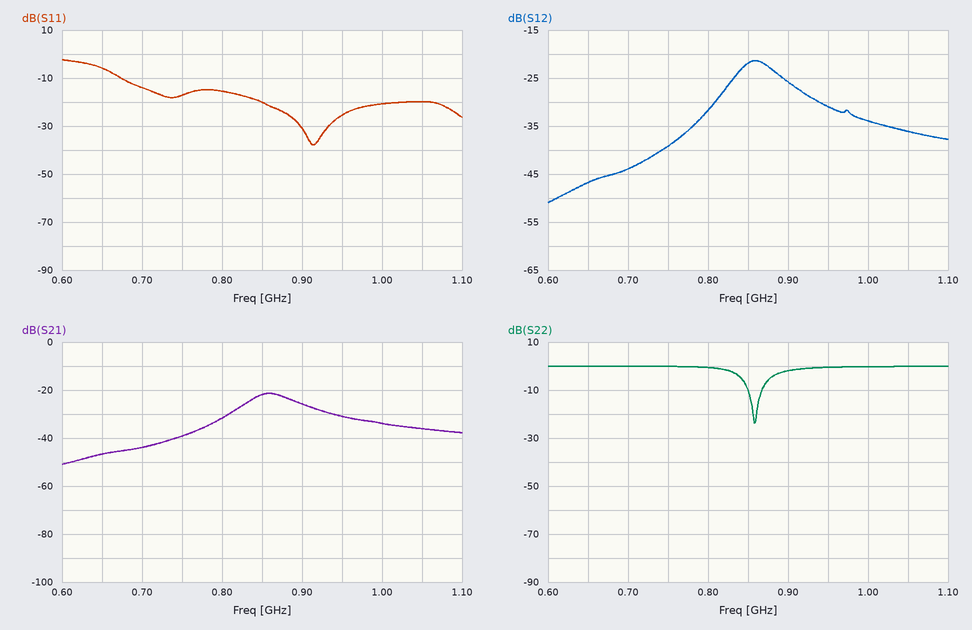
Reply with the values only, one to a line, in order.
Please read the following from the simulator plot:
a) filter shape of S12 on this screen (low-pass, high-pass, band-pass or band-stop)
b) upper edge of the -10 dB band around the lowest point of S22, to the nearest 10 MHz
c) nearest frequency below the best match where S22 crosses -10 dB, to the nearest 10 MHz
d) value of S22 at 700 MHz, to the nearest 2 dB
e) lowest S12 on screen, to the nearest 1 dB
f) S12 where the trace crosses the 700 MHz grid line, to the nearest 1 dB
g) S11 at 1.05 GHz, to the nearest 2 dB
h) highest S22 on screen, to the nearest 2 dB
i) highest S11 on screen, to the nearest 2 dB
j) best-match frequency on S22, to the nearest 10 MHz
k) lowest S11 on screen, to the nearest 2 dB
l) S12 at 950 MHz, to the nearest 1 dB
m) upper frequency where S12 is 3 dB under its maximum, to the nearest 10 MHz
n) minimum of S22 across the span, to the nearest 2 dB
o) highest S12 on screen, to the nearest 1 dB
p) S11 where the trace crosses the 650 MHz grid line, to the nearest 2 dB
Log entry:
band-pass
870 MHz
850 MHz
0 dB
-51 dB
-44 dB
-20 dB
0 dB
-2 dB
860 MHz
-38 dB
-31 dB
890 MHz
-24 dB
-21 dB
-6 dB
